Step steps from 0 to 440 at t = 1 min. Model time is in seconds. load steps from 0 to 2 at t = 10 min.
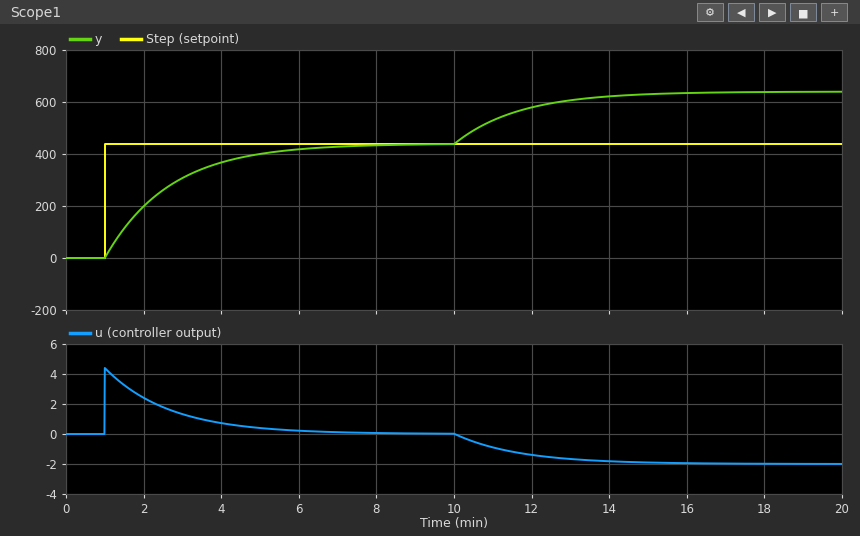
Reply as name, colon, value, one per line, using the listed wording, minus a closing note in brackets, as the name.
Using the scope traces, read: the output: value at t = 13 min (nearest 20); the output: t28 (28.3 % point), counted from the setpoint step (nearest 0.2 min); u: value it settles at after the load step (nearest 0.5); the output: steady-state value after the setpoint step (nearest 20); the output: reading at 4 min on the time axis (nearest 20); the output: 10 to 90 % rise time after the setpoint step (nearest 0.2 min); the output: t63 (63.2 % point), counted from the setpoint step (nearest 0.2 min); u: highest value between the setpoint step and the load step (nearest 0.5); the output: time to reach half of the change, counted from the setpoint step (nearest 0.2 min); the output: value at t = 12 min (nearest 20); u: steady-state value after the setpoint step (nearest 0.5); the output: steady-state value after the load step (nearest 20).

the output: value at t = 13 min: 600
the output: t28 (28.3 % point), counted from the setpoint step: 0.6 min
u: value it settles at after the load step: -2.0
the output: steady-state value after the setpoint step: 440
the output: reading at 4 min on the time axis: 360
the output: 10 to 90 % rise time after the setpoint step: 3.6 min
the output: t63 (63.2 % point), counted from the setpoint step: 1.6 min
u: highest value between the setpoint step and the load step: 4.5
the output: time to reach half of the change, counted from the setpoint step: 1.2 min
the output: value at t = 12 min: 580
u: steady-state value after the setpoint step: 0.0
the output: steady-state value after the load step: 640
